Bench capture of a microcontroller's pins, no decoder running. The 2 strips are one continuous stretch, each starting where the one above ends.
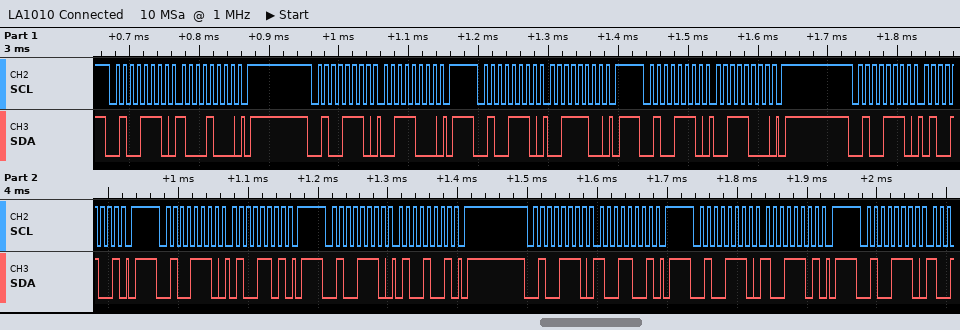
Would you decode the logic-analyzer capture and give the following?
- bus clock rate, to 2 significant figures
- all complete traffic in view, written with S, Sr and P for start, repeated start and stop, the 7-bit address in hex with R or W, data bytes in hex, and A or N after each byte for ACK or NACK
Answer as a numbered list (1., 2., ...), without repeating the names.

1. 100 kHz
2. S 27W A 88 A P S 27W A 38 A P S 27W A 3C A P S 27W A 38 A P S 27W A 49 A P S 27W A 4D A P S 27W A 49 A P S 27W A 99 A P S 27W A 9D A P S 27W A
